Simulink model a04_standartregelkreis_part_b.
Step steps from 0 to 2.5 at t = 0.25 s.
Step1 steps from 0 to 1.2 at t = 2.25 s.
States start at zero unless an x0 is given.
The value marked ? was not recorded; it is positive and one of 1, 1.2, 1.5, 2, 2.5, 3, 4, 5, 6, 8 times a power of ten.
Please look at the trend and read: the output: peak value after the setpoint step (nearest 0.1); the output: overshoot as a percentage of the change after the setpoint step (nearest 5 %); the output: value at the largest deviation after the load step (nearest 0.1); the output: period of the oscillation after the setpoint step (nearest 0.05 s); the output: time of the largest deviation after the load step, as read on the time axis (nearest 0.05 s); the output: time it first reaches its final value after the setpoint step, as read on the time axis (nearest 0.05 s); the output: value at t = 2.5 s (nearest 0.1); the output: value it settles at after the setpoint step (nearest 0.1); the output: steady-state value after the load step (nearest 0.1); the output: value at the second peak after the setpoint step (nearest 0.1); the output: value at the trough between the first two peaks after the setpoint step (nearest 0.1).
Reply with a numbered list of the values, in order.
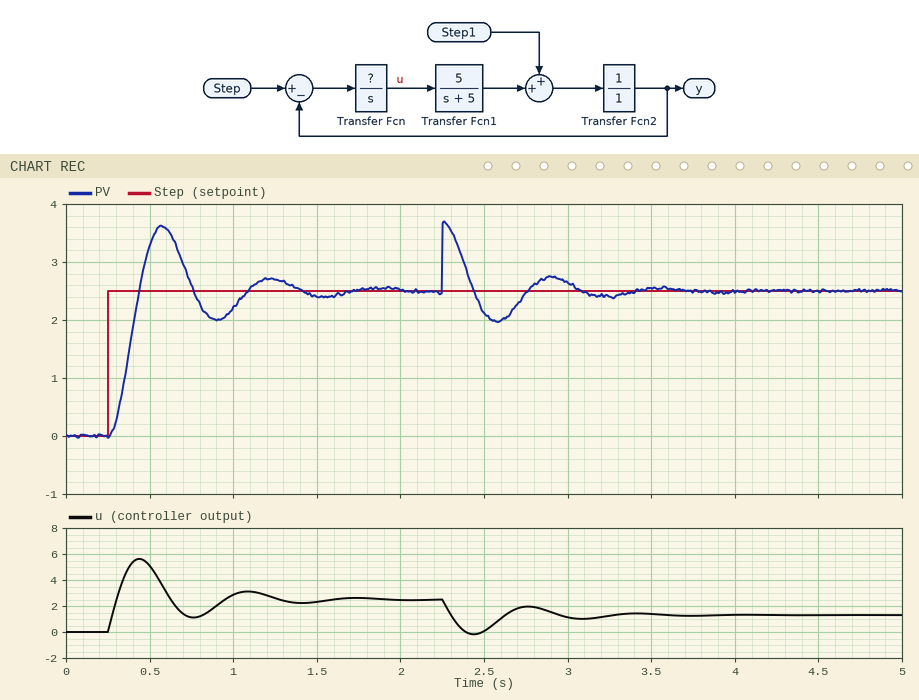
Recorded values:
1. 3.6
2. 45 %
3. 3.7
4. 0.65 s
5. 2.25 s
6. 0.45 s
7. 2.1
8. 2.5
9. 2.5
10. 2.7
11. 2.0
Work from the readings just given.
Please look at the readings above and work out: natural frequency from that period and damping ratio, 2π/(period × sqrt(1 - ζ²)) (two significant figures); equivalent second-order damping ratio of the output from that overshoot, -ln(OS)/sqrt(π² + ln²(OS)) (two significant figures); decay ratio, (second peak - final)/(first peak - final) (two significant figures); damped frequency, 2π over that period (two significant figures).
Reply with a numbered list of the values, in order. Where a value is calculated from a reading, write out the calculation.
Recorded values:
1. 2π / (0.65 × sqrt(1 - 0.25²)) = 10.0 rad/s
2. ln(0.45) = -0.799; 0.799 / sqrt(9.870 + 0.638) = 0.25
3. (2.7 - 2.5) / (3.6 - 2.5) = 0.18
4. 2π / 0.65 = 9.7 rad/s
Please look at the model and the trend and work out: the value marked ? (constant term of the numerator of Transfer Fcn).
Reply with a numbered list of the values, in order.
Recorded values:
1. 20
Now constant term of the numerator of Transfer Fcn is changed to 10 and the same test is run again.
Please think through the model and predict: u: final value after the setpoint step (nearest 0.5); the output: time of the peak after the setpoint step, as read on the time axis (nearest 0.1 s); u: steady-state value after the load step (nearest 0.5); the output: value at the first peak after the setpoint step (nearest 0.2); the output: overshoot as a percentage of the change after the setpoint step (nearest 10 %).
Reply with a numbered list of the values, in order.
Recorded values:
1. 2.5
2. 0.7 s
3. 1.5
4. 3.2
5. 30 %
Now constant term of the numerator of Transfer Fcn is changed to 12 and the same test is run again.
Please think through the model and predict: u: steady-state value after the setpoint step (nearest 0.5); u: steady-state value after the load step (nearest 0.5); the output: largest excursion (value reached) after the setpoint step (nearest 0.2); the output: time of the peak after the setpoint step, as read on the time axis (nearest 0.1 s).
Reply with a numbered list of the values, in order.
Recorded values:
1. 2.5
2. 1.5
3. 3.4
4. 0.7 s
